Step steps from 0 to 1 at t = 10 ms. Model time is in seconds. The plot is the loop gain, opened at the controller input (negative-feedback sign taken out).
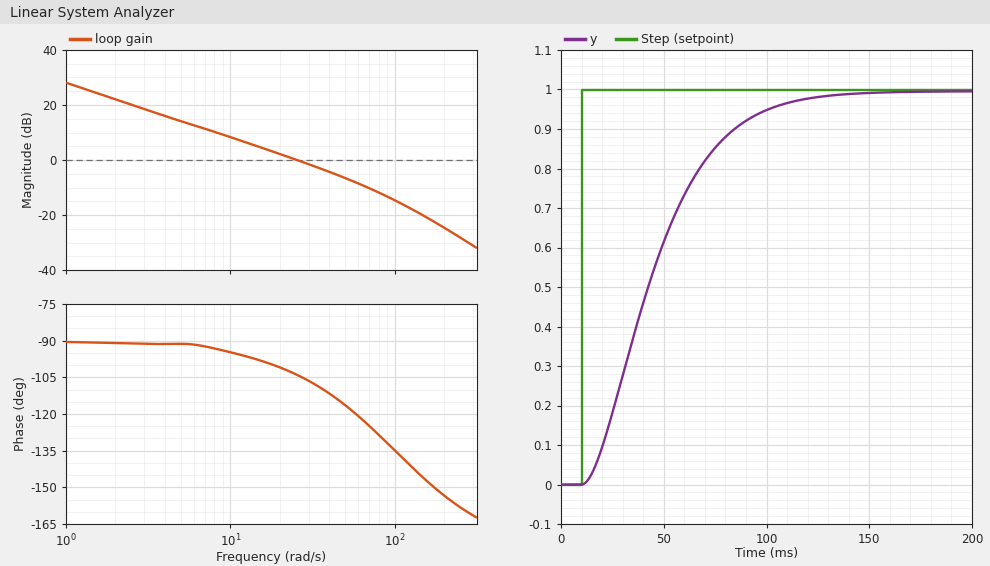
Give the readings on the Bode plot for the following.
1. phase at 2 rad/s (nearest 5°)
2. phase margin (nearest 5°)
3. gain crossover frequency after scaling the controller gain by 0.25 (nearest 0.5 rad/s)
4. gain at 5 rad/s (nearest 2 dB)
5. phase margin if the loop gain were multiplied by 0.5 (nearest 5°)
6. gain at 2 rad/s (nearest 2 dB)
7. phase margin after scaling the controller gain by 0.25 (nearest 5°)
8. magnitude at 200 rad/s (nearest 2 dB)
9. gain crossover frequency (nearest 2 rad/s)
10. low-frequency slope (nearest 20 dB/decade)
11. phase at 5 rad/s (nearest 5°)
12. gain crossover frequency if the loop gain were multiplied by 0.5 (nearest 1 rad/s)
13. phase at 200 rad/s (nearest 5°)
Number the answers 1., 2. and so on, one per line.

1. -90°
2. 75°
3. 6.5 rad/s
4. 14 dB
5. 85°
6. 22 dB
7. 90°
8. -24 dB
9. 26 rad/s
10. -20 dB/decade
11. -90°
12. 13 rad/s
13. -155°
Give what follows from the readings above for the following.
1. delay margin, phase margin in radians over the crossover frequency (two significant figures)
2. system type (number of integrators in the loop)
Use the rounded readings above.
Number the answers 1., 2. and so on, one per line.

1. 0.050 s
2. 1
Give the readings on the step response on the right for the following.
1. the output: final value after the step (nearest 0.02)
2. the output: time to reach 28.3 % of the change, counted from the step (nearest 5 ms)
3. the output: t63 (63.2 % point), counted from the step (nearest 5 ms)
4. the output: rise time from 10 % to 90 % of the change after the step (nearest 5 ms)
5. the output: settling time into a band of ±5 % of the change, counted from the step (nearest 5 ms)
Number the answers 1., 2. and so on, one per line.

1. 1.00
2. 20 ms
3. 40 ms
4. 65 ms
5. 90 ms
